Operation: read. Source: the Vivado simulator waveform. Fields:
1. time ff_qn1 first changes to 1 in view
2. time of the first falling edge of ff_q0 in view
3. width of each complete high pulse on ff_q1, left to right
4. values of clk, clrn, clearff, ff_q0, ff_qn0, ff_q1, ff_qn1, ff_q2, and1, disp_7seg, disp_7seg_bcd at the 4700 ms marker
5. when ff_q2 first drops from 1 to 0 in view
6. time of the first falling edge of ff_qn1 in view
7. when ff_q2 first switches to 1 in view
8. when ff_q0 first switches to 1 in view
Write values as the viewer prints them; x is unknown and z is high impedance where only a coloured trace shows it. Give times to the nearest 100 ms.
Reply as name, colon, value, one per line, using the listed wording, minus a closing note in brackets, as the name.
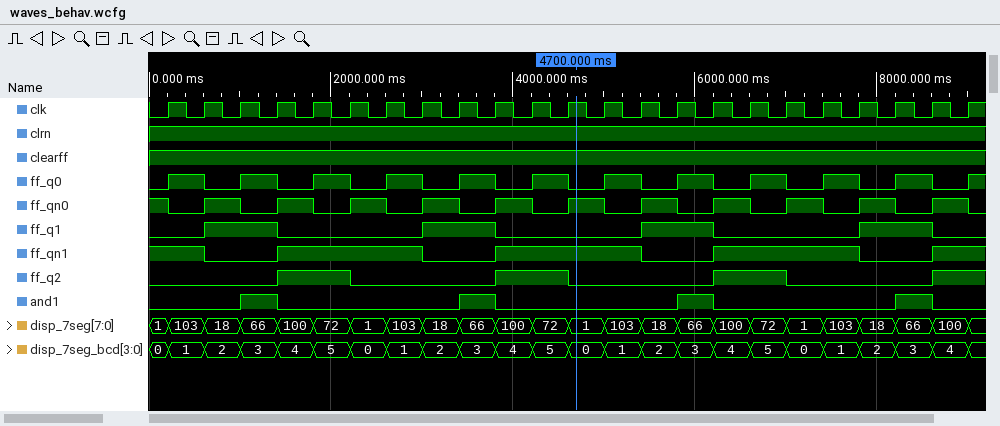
time ff_qn1 first changes to 1 in view: 1400 ms
time of the first falling edge of ff_q0 in view: 600 ms
width of each complete high pulse on ff_q1, left to right: 800 ms, 800 ms, 800 ms, 800 ms
values of clk, clrn, clearff, ff_q0, ff_qn0, ff_q1, ff_qn1, ff_q2, and1, disp_7seg, disp_7seg_bcd at the 4700 ms marker: clk=1, clrn=1, clearff=1, ff_q0=0, ff_qn0=1, ff_q1=0, ff_qn1=1, ff_q2=0, and1=0, disp_7seg=1, disp_7seg_bcd=0
when ff_q2 first drops from 1 to 0 in view: 2200 ms
time of the first falling edge of ff_qn1 in view: 600 ms
when ff_q2 first switches to 1 in view: 1400 ms
when ff_q0 first switches to 1 in view: 200 ms
